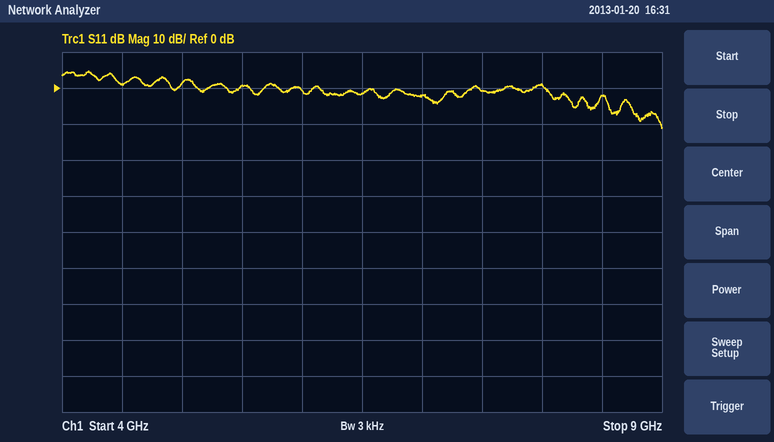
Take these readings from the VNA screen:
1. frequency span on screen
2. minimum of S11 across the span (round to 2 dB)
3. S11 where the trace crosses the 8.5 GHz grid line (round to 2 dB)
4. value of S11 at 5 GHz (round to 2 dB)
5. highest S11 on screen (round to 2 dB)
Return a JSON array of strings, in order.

["5 GHz", "-12 dB", "-2 dB", "2 dB", "4 dB"]
